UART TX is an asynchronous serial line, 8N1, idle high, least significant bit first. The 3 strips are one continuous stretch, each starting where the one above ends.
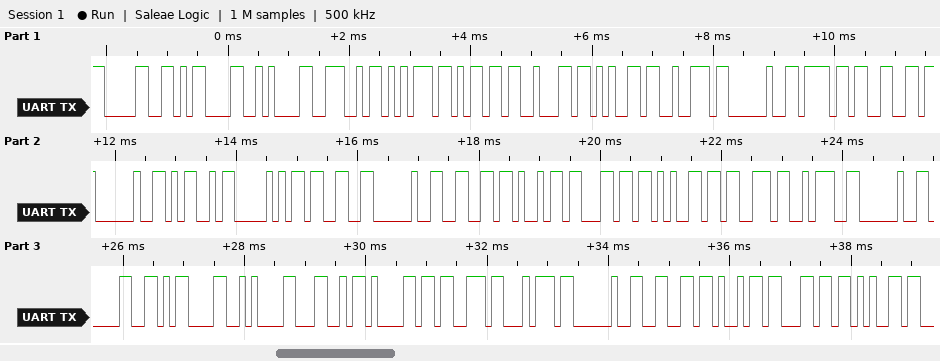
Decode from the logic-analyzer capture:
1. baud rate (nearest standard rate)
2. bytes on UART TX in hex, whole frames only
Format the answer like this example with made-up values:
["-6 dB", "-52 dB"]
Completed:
["9600 baud", "30 0D 0A 4E 75 6D 62 65 72 20 6F 66 20 4D 50 33 20 66 69 6C 65 73 3A 20 30 0D 0A 4C 61 73 74 20 66 69 6C 65"]
